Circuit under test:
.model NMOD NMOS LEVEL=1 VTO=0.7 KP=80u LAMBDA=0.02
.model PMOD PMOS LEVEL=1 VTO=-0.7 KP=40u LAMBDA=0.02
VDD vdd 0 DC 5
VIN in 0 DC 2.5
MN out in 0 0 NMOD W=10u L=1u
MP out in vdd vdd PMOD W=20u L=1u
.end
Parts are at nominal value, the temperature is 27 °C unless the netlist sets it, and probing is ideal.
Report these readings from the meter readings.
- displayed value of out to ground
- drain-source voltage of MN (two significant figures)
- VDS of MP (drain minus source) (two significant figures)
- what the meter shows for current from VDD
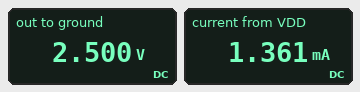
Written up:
2.500 V
2.5 V
-2.5 V
1.361 mA
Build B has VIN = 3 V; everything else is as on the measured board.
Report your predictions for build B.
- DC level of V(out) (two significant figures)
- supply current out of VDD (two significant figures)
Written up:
440 mV
740 µA
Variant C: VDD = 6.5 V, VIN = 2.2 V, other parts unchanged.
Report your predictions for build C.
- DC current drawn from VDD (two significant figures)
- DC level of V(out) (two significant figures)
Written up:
1.0 mA
6.1 V
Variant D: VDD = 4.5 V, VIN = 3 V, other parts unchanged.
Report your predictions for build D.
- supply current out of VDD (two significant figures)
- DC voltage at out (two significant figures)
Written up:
280 µA
160 mV
